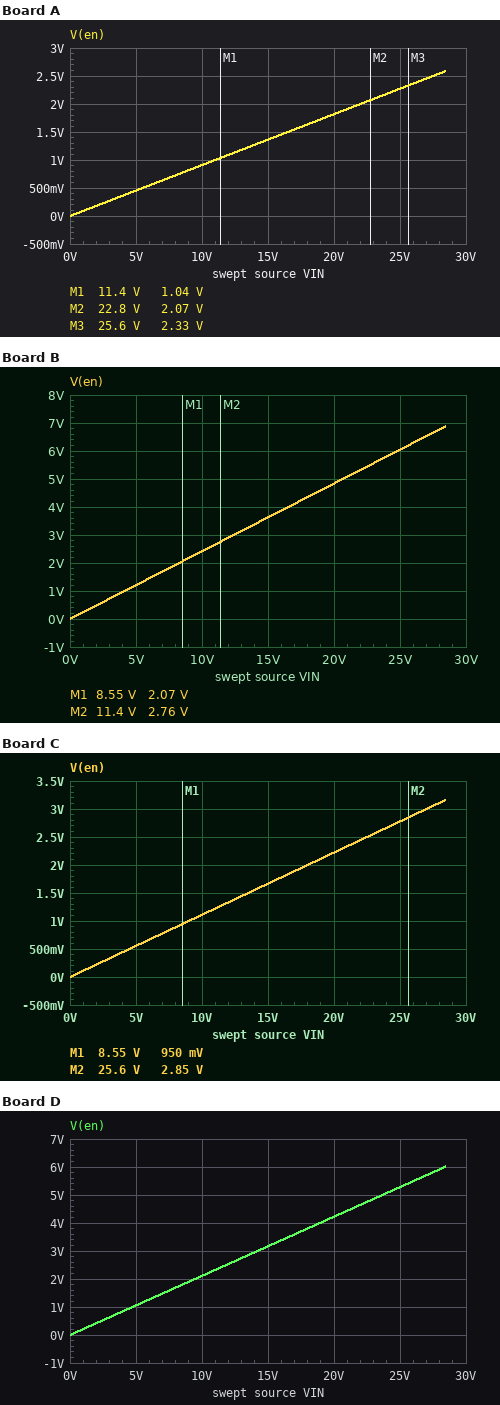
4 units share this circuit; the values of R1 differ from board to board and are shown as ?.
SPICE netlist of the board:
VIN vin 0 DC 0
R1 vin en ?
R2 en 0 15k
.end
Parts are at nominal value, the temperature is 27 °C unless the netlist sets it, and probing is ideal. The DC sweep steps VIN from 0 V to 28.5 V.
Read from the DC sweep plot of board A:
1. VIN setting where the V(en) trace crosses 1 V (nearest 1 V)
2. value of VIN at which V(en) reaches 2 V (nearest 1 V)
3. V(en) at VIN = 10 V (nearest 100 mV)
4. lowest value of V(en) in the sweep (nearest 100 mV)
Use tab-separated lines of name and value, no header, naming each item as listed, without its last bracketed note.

VIN setting where the V(en) trace crosses 1 V	11 V
value of VIN at which V(en) reaches 2 V	22 V
V(en) at VIN = 10 V	900 mV
lowest value of V(en) in the sweep	0 V
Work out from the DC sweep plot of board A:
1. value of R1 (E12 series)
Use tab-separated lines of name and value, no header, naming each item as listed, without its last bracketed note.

value of R1	150 kΩ
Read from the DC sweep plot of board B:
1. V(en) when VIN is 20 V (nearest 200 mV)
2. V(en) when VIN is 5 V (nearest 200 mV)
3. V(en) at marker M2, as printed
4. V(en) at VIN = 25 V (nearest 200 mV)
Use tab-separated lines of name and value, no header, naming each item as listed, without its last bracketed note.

V(en) when VIN is 20 V	4.8 V
V(en) when VIN is 5 V	1.2 V
V(en) at marker M2, as printed	2.76 V
V(en) at VIN = 25 V	6.0 V
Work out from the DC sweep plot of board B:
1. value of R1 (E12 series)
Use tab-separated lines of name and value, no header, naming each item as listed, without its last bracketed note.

value of R1	47 kΩ
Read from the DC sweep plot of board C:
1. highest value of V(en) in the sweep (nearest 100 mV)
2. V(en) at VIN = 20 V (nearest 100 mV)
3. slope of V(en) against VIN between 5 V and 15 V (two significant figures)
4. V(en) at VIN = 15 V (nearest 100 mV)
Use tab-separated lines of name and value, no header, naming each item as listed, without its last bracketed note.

highest value of V(en) in the sweep	3.2 V
V(en) at VIN = 20 V	2.2 V
slope of V(en) against VIN between 5 V and 15 V	0.11 V/V
V(en) at VIN = 15 V	1.7 V
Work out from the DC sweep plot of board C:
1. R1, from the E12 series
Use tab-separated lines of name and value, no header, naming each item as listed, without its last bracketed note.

R1, from the E12 series	120 kΩ
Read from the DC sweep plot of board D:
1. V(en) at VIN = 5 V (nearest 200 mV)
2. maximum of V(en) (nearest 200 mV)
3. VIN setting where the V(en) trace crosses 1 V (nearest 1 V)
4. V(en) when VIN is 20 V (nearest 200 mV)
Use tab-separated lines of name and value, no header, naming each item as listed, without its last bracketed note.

V(en) at VIN = 5 V	1.0 V
maximum of V(en)	6.0 V
VIN setting where the V(en) trace crosses 1 V	5 V
V(en) when VIN is 20 V	4.2 V
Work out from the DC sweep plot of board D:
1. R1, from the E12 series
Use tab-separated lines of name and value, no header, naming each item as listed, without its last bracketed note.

R1, from the E12 series	56 kΩ
